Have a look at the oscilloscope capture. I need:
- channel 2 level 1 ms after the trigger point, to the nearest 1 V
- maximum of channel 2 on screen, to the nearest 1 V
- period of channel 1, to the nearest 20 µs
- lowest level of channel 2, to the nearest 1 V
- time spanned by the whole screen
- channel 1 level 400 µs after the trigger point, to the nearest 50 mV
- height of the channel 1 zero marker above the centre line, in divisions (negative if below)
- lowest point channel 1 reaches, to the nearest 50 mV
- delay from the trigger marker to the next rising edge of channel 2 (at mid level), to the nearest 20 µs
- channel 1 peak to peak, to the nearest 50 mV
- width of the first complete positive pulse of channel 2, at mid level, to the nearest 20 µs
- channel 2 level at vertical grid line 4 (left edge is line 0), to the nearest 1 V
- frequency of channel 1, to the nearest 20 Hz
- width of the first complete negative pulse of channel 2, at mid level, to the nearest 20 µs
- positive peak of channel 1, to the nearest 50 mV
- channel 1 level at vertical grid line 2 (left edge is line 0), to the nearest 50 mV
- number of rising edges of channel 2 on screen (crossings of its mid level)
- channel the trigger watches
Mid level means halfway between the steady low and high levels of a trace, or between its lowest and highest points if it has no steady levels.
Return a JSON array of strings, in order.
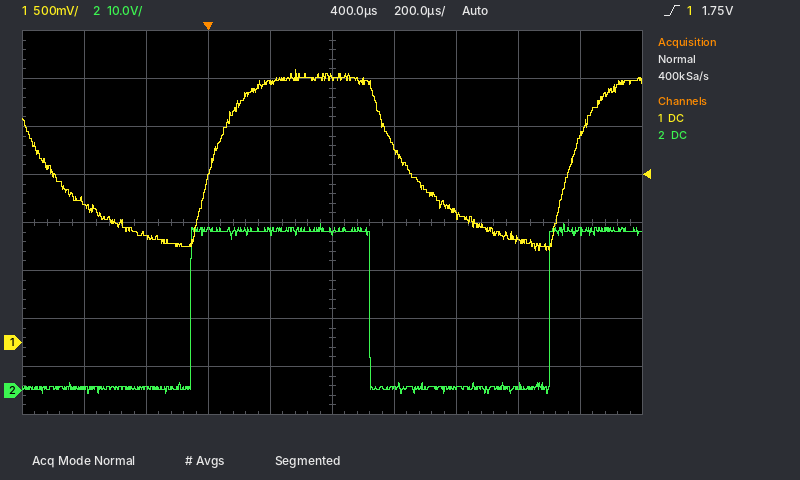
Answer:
["1 V", "35 V", "1.16 ms", "-1 V", "2 ms", "2.75 V", "-2.5 div", "950 mV", "1.10 ms", "1.90 V", "580 µs", "33 V", "860 Hz", "580 µs", "2.85 V", "1.10 V", "2", "channel 1"]
